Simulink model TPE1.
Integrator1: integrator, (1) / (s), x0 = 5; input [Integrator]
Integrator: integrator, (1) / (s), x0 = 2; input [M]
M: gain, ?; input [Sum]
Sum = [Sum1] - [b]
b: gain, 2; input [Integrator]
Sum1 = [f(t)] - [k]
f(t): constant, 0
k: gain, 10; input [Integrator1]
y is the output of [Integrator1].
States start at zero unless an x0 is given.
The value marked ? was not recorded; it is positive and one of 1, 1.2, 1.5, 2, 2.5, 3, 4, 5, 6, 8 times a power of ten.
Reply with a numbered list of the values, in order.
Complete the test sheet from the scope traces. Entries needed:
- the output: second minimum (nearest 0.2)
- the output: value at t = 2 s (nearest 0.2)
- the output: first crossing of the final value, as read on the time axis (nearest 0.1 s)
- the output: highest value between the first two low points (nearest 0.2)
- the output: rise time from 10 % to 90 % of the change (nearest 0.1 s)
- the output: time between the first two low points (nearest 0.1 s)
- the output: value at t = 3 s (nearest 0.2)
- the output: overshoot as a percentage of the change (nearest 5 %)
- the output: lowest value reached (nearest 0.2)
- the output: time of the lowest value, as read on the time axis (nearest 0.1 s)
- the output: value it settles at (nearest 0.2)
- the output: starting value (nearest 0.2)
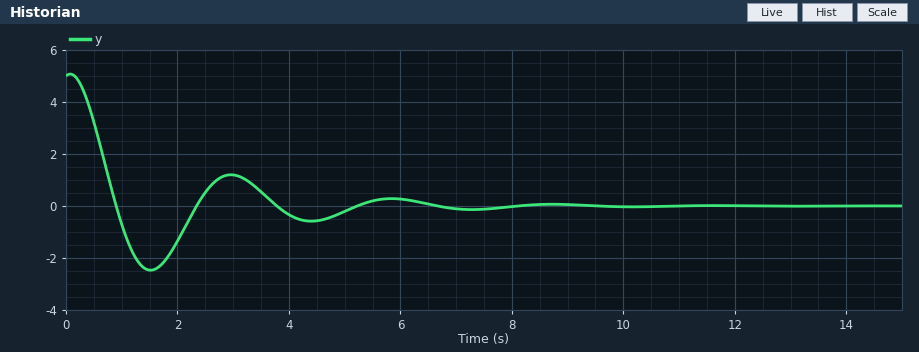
1. -0.6
2. -1.4
3. 0.9 s
4. 1.2
5. 0.5 s
6. 2.9 s
7. 1.2
8. 50 %
9. -2.4
10. 1.5 s
11. 0.0
12. 5.0
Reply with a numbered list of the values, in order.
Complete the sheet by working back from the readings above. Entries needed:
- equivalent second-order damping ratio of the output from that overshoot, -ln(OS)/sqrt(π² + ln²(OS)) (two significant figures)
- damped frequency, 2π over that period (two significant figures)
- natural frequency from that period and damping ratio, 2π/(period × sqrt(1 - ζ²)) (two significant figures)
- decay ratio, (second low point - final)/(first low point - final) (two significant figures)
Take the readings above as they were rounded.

1. 0.22
2. 2.2 rad/s
3. 2.2 rad/s
4. 0.25
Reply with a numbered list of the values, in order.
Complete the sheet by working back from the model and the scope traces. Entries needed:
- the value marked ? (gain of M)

1. 0.5
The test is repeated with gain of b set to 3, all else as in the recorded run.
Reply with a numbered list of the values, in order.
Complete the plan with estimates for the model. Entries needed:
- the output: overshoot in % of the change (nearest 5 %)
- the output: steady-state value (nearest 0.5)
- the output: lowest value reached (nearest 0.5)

1. 35 %
2. 0.0
3. -1.5
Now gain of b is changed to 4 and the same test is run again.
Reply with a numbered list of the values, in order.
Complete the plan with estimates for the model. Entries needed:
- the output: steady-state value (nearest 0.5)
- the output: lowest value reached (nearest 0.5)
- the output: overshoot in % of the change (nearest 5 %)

1. 0.0
2. -1.0
3. 20 %
